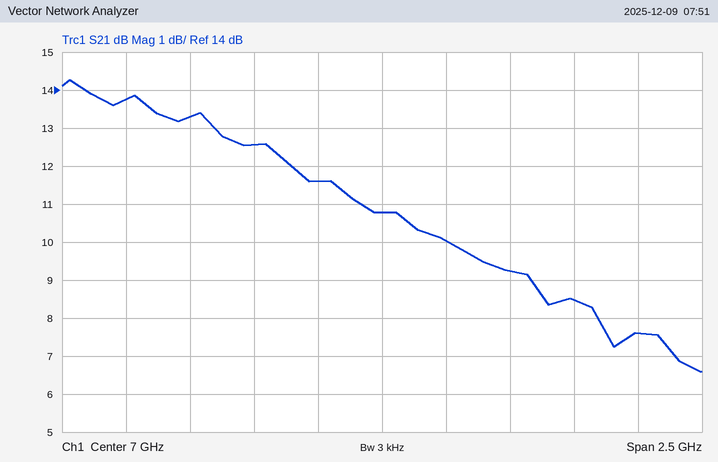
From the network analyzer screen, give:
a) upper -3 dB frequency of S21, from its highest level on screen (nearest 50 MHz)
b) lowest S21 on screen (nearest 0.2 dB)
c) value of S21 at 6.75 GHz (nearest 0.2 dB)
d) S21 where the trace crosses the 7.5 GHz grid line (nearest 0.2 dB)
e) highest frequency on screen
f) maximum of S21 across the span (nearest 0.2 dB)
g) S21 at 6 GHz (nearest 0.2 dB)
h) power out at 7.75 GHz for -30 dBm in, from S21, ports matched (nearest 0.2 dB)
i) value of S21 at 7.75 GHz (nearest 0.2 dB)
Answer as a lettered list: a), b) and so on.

a) 6.85 GHz
b) 6.6 dB
c) 11.6 dB
d) 9.2 dB
e) 8.25 GHz
f) 14.2 dB
g) 13.8 dB
h) -21.6 dBm
i) 8.4 dB
